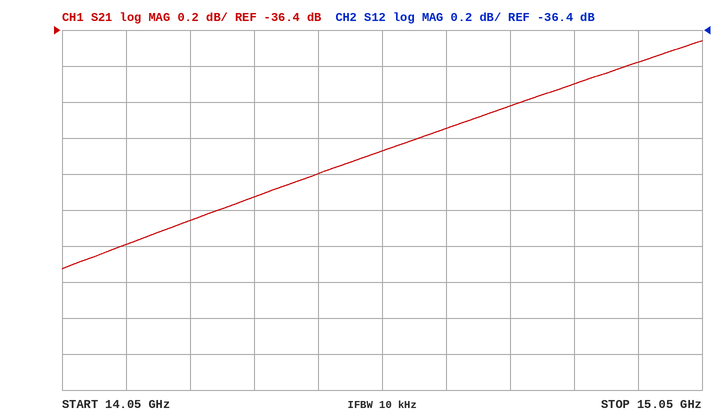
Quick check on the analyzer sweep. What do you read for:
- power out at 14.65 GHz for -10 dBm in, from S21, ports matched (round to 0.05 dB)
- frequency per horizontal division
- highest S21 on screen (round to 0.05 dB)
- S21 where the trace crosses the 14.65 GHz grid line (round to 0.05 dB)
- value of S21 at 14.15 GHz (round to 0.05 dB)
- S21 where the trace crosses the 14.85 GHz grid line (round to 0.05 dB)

-46.95 dBm
100 MHz
-36.45 dB
-36.95 dB
-37.60 dB
-36.70 dB
